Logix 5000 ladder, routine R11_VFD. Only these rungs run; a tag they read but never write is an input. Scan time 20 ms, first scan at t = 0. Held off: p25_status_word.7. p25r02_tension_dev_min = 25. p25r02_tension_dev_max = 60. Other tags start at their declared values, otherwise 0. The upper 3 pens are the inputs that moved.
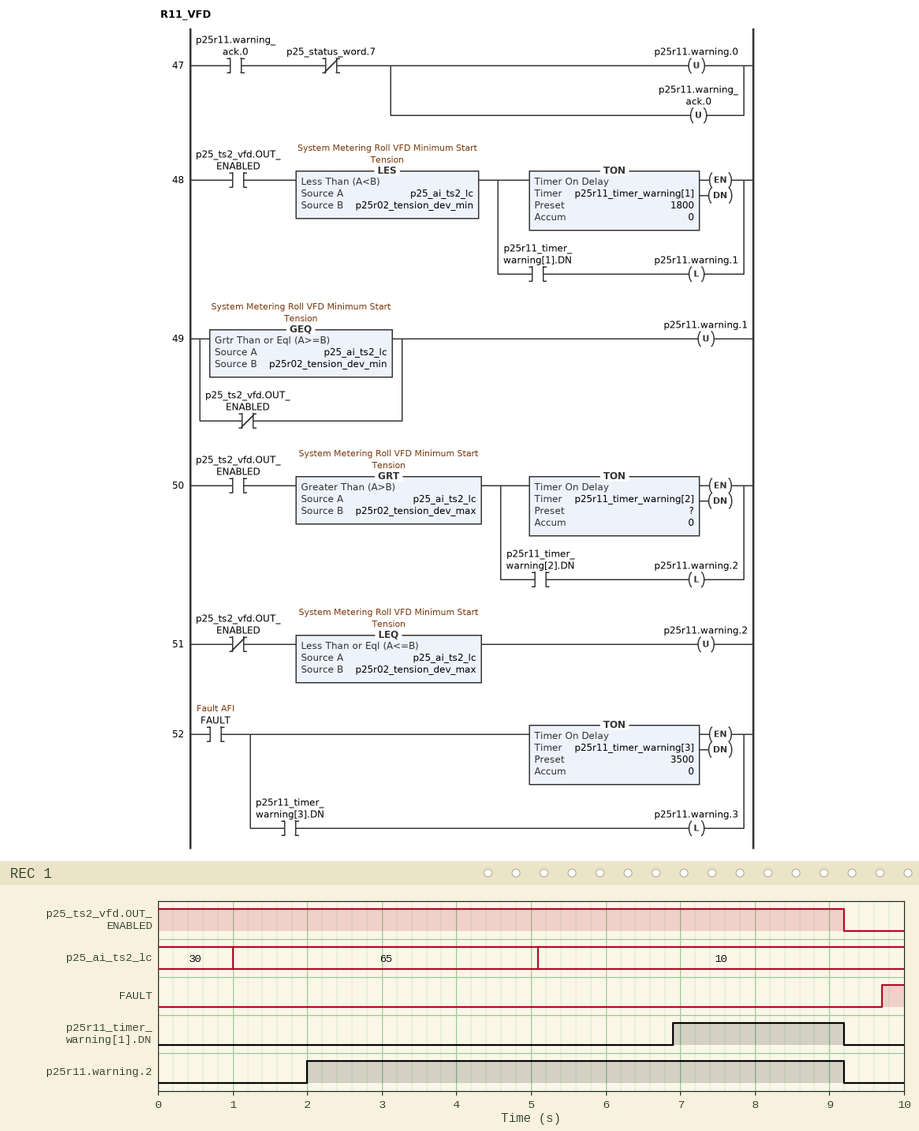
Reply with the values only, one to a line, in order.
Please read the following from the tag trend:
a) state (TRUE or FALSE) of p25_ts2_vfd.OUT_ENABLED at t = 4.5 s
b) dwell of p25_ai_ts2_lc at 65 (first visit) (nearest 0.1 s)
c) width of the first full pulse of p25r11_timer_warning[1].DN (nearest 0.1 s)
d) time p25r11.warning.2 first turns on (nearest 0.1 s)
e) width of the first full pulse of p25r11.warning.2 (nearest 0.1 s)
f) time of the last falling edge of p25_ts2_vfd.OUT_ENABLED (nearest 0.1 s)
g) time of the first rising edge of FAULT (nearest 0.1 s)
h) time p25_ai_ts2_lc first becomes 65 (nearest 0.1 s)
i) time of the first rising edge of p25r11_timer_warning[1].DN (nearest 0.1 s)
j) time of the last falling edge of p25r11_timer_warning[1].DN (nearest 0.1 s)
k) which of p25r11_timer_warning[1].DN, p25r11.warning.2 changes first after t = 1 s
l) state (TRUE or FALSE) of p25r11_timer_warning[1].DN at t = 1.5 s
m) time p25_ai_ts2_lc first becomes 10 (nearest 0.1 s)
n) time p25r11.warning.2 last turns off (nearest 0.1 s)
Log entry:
TRUE
4.1 s
2.3 s
2.0 s
7.2 s
9.2 s
9.7 s
1.0 s
6.9 s
9.2 s
p25r11.warning.2
FALSE
5.1 s
9.2 s
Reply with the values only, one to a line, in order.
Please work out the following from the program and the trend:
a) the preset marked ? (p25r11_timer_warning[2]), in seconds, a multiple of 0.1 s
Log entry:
1.0 s
